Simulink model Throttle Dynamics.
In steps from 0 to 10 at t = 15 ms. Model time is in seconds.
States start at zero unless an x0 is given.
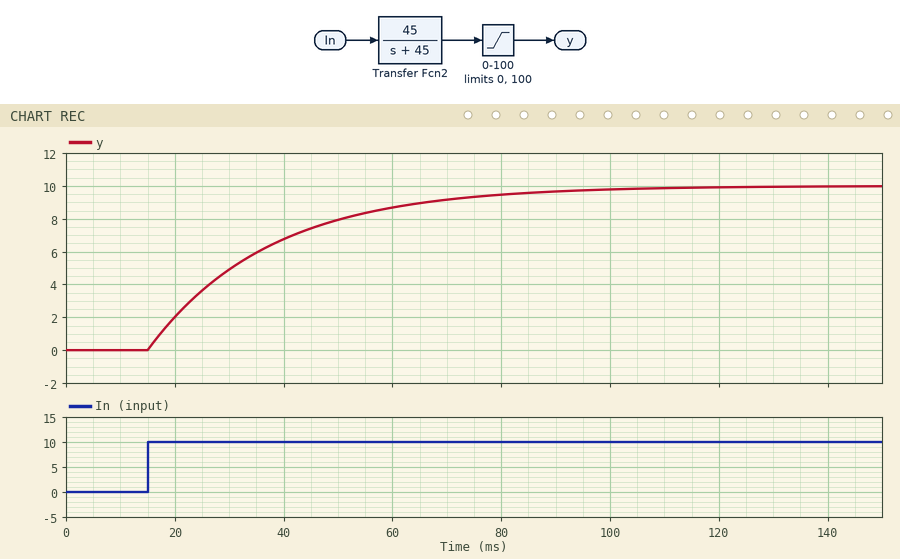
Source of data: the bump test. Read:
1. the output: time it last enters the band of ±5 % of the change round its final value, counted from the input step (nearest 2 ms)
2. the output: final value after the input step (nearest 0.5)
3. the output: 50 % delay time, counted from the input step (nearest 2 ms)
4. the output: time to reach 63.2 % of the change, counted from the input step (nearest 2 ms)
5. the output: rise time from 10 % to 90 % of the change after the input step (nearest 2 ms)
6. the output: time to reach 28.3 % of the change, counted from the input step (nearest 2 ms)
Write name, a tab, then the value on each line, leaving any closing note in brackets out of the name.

the output: time it last enters the band of ±5 % of the change round its final value, counted from the input step	66 ms
the output: final value after the input step	10.0
the output: 50 % delay time, counted from the input step	16 ms
the output: time to reach 63.2 % of the change, counted from the input step	22 ms
the output: rise time from 10 % to 90 % of the change after the input step	48 ms
the output: time to reach 28.3 % of the change, counted from the input step	8 ms
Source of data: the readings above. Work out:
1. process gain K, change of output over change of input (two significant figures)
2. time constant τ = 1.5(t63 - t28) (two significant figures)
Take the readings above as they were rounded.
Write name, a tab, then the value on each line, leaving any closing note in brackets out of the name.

process gain K, change of output over change of input	1.0
time constant τ = 1.5(t63 - t28)	21 ms
